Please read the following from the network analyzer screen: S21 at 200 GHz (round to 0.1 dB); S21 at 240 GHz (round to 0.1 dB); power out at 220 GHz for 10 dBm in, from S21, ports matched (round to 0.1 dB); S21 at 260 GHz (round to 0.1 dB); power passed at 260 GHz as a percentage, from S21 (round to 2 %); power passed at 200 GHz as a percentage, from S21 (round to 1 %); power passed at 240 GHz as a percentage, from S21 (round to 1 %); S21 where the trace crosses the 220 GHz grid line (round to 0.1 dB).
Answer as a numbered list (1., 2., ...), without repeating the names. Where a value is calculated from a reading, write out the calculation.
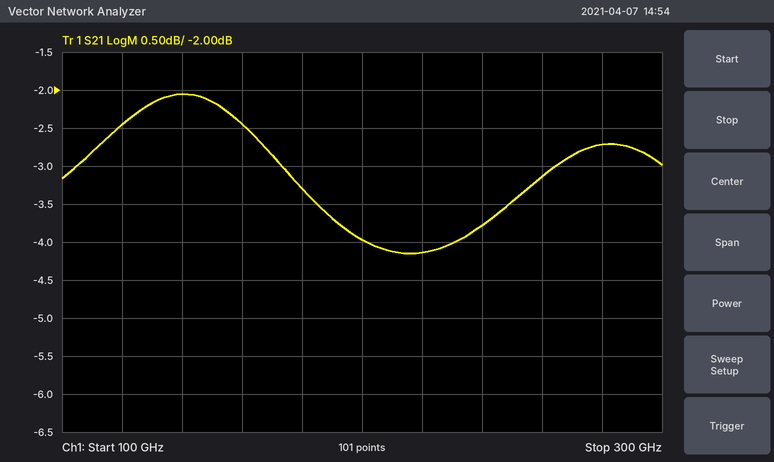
1. -4.0 dB
2. -3.8 dB
3. 10 dBm + (-4.1 dB) = 5.9 dBm
4. -3.1 dB
5. 10^(-3.1/10) ≈ 49.0 %, so 48 % to the nearest 2 %
6. 10^(-4/10) ≈ 40 %
7. 10^(-3.8/10) ≈ 42 %
8. -4.1 dB
